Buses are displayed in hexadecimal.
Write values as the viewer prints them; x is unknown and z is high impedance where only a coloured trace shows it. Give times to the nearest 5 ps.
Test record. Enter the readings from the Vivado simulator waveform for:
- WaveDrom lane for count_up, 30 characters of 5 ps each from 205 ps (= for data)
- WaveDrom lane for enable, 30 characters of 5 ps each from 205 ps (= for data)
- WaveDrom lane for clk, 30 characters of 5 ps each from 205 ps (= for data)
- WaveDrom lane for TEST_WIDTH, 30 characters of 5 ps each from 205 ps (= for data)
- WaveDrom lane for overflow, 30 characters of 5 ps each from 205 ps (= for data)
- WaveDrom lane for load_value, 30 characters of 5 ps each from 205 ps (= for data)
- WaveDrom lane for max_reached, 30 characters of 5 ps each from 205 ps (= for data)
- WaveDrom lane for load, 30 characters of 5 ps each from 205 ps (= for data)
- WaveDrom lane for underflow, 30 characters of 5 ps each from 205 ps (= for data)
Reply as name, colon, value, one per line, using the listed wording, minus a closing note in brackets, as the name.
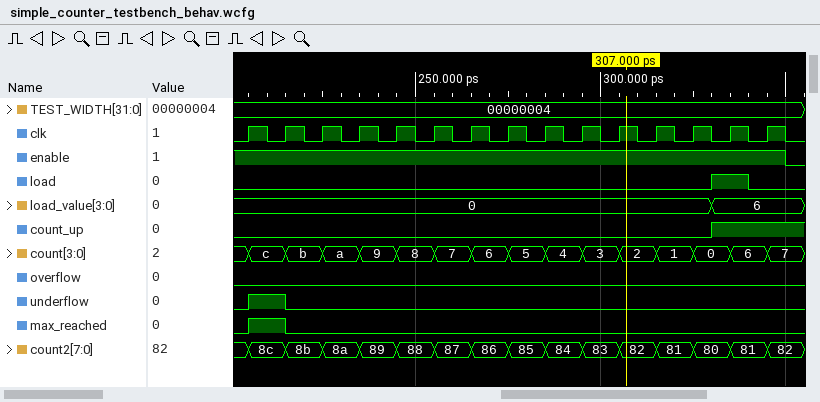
WaveDrom lane for count_up, 30 characters of 5 ps each from 205 ps: {name: 'count_up', wave: '0........................1....'}
WaveDrom lane for enable, 30 characters of 5 ps each from 205 ps: {name: 'enable', wave: '1............................0'}
WaveDrom lane for clk, 30 characters of 5 ps each from 205 ps: {name: 'clk', wave: '101010101010101010101010101010'}
WaveDrom lane for TEST_WIDTH, 30 characters of 5 ps each from 205 ps: {name: 'TEST_WIDTH', wave: '=.............................', data: '00000004'}
WaveDrom lane for overflow, 30 characters of 5 ps each from 205 ps: {name: 'overflow', wave: '0.............................'}
WaveDrom lane for load_value, 30 characters of 5 ps each from 205 ps: {name: 'load_value', wave: '=........................=....', data: '0 6'}
WaveDrom lane for max_reached, 30 characters of 5 ps each from 205 ps: {name: 'max_reached', wave: '1.0...........................'}
WaveDrom lane for load, 30 characters of 5 ps each from 205 ps: {name: 'load', wave: '0........................1.0..'}
WaveDrom lane for underflow, 30 characters of 5 ps each from 205 ps: {name: 'underflow', wave: '1.0...........................'}
